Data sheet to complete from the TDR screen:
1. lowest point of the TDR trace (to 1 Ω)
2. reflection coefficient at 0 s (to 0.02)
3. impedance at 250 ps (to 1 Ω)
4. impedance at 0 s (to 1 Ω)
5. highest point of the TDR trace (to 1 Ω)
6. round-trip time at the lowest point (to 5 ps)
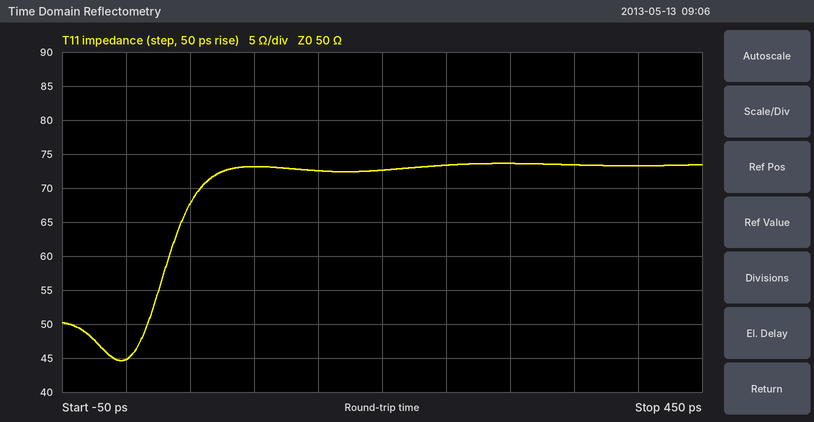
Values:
45 Ω
-0.06
73 Ω
45 Ω
74 Ω
-5 ps
